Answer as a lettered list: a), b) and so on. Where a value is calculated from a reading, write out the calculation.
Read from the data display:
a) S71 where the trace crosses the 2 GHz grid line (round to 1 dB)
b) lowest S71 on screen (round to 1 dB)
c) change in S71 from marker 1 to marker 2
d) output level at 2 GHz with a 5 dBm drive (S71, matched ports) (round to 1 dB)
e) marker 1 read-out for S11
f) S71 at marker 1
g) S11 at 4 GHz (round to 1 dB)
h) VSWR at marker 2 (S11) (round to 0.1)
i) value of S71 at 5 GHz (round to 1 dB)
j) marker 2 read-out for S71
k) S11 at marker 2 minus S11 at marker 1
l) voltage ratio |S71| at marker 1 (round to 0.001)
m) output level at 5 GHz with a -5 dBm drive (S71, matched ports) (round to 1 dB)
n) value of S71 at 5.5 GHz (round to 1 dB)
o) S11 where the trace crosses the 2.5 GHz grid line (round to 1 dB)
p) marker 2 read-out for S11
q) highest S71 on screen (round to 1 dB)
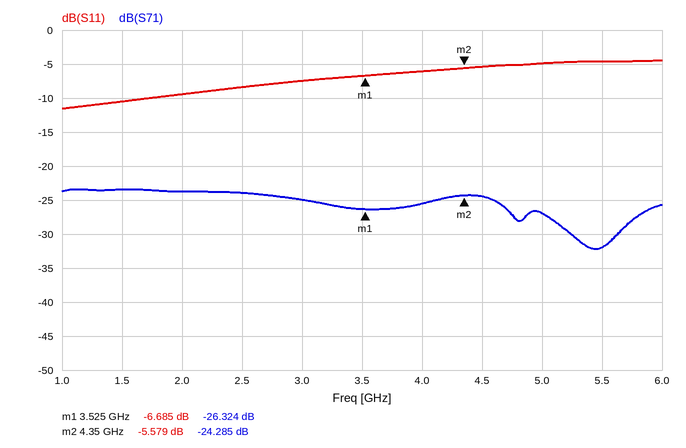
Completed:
a) -24 dB
b) -32 dB
c) -24.285 − (-26.324) = 2.039 dB
d) 5 dBm + (-24 dB) = -19 dBm
e) -6.685 dB
f) -26.324 dB
g) -6 dB
h) (1 + 0.5261)/(1 − 0.5261) ≈ 3.2
i) -27 dB
j) -24.285 dB
k) -5.579 − (-6.685) = 1.106 dB
l) 10^(-26.324/20) ≈ 0.048
m) -5 dBm + (-27 dB) = -32 dBm
n) -32 dB
o) -8 dB
p) -5.579 dB
q) -23 dB
